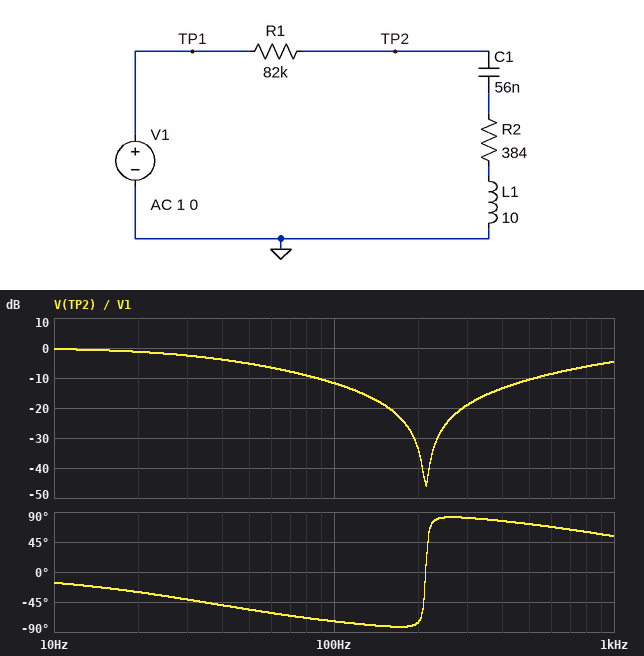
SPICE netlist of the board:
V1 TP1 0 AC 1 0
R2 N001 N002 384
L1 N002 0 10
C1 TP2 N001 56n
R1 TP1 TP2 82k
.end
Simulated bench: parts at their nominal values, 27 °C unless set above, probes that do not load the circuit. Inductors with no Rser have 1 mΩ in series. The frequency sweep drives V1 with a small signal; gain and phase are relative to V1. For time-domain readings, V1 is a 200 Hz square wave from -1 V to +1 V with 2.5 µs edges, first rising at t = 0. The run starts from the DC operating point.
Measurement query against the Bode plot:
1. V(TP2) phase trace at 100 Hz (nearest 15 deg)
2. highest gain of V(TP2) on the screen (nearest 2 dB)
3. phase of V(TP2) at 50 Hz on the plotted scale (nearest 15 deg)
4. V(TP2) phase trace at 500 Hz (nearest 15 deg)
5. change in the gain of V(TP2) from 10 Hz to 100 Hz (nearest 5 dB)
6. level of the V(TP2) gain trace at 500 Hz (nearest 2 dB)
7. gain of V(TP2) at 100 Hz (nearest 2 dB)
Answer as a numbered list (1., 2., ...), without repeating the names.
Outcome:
1. -75 deg
2. 0 dB
3. -60 deg
4. 75 deg
5. -10 dB
6. -10 dB
7. -12 dB
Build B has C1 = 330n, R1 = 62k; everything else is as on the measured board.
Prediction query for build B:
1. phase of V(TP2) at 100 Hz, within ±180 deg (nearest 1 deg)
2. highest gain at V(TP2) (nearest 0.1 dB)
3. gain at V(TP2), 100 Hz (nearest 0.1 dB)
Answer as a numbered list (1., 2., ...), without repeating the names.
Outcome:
1. 74 deg
2. 0 dB
3. -32.3 dB
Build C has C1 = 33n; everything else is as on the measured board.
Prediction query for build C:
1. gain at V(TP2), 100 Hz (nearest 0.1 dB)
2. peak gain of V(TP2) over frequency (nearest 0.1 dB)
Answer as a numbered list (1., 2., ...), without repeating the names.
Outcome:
1. -6.9 dB
2. 0 dB
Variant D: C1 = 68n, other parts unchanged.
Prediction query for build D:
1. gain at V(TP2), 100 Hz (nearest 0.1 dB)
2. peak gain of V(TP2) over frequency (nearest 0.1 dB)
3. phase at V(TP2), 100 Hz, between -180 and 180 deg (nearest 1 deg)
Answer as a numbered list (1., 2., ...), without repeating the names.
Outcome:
1. -13.8 dB
2. 0 dB
3. -77 deg
